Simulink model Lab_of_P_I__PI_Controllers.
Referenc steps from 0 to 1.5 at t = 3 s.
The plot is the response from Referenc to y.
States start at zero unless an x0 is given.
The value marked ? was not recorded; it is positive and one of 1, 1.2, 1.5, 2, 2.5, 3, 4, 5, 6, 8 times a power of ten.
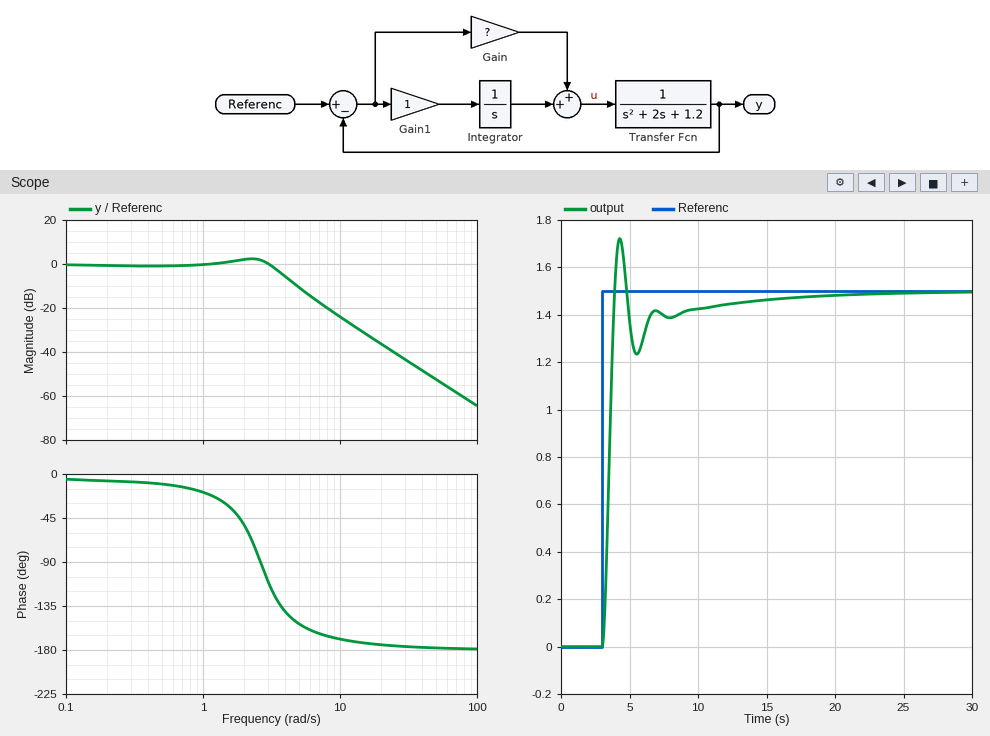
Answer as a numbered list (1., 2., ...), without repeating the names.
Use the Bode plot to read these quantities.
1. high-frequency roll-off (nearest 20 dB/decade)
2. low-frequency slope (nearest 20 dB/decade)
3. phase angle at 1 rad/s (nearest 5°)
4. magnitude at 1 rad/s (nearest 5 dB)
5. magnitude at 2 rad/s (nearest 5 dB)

1. -40 dB/decade
2. 0 dB/decade
3. -20°
4. 0 dB
5. 0 dB
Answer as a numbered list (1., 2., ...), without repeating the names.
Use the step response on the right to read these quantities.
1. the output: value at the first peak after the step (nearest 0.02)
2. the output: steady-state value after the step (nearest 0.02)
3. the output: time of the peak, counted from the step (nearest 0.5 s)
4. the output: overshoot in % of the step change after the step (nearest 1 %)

1. 1.72
2. 1.50
3. 1.5 s
4. 15 %
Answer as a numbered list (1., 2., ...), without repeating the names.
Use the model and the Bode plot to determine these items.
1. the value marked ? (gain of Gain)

1. 6
